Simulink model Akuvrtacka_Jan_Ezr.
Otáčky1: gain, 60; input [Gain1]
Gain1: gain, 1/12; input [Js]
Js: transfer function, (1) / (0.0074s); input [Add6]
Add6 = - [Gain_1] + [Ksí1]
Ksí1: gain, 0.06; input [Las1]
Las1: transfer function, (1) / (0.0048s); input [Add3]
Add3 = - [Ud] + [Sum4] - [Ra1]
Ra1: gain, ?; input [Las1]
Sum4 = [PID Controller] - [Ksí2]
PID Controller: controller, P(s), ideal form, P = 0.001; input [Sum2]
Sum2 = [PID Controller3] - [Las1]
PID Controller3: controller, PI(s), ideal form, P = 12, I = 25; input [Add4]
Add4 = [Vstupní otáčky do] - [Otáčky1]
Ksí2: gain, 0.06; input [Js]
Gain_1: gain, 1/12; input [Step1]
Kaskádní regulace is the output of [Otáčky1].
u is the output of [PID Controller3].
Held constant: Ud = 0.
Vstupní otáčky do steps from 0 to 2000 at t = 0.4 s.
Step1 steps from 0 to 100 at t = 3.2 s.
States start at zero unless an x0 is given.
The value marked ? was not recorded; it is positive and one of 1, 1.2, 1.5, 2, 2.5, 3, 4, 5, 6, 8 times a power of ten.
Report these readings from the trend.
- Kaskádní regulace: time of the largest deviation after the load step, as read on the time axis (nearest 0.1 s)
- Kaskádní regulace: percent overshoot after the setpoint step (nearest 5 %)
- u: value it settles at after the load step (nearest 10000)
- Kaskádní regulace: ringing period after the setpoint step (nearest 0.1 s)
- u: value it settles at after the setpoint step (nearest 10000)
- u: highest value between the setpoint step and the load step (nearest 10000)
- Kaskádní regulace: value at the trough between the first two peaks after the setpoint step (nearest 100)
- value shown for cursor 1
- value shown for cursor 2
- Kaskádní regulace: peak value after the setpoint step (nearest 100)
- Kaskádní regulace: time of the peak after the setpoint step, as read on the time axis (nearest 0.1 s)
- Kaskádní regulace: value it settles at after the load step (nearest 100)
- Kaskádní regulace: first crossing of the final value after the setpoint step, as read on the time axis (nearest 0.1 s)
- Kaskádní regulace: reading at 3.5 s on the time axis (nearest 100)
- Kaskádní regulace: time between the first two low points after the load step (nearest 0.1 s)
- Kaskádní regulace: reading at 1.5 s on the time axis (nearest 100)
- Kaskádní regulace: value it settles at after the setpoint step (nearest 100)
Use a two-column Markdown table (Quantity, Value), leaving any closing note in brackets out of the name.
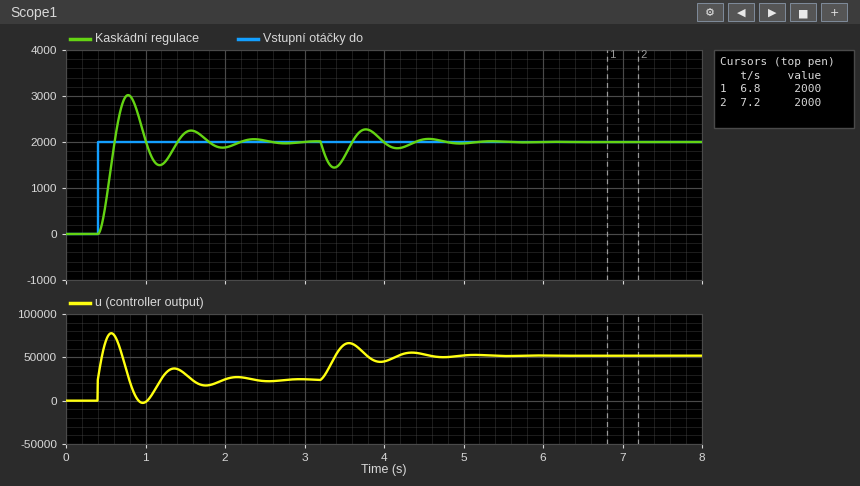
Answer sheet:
| Quantity | Value |
|---|---|
| Kaskádní regulace: time of the largest deviation after the load step, as read on the time axis | 3.4 s |
| Kaskádní regulace: percent overshoot after the setpoint step | 50 % |
| u: value it settles at after the load step | 50000 |
| Kaskádní regulace: ringing period after the setpoint step | 0.8 s |
| u: value it settles at after the setpoint step | 20000 |
| u: highest value between the setpoint step and the load step | 80000 |
| Kaskádní regulace: value at the trough between the first two peaks after the setpoint step | 1500 |
| value shown for cursor 1 | 2000 |
| value shown for cursor 2 | 2000 |
| Kaskádní regulace: peak value after the setpoint step | 3000 |
| Kaskádní regulace: time of the peak after the setpoint step, as read on the time axis | 0.8 s |
| Kaskádní regulace: value it settles at after the load step | 2000 |
| Kaskádní regulace: first crossing of the final value after the setpoint step, as read on the time axis | 0.6 s |
| Kaskádní regulace: reading at 3.5 s on the time axis | 1700 |
| Kaskádní regulace: time between the first two low points after the load step | 0.8 s |
| Kaskádní regulace: reading at 1.5 s on the time axis | 2200 |
| Kaskádní regulace: value it settles at after the setpoint step | 2000 |
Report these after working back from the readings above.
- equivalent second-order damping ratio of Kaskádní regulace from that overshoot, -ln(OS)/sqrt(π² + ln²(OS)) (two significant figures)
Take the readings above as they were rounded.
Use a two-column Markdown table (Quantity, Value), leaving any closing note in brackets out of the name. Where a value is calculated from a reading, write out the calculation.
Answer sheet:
| Quantity | Value |
|---|---|
| equivalent second-order damping ratio of Kaskádní regulace from that overshoot, -ln(OS)/sqrt(π² + ln²(OS)) | ln(0.5) = -0.693; 0.693 / sqrt(9.870 + 0.480) = 0.22 |
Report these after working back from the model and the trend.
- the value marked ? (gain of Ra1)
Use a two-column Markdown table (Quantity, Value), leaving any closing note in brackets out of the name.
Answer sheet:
| Quantity | Value |
|---|---|
| the value marked ? | 0.2 |
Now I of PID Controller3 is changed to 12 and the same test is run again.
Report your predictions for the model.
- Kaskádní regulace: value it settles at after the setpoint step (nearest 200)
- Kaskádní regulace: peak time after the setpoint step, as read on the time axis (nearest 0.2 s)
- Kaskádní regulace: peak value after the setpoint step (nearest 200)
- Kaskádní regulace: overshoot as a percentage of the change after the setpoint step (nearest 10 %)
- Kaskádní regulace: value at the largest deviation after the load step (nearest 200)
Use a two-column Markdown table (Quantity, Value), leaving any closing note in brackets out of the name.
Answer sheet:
| Quantity | Value |
|---|---|
| Kaskádní regulace: value it settles at after the setpoint step | 2000 |
| Kaskádní regulace: peak time after the setpoint step, as read on the time axis | 1.0 s |
| Kaskádní regulace: peak value after the setpoint step | 2600 |
| Kaskádní regulace: overshoot as a percentage of the change after the setpoint step | 30 % |
| Kaskádní regulace: value at the largest deviation after the load step | 1400 |
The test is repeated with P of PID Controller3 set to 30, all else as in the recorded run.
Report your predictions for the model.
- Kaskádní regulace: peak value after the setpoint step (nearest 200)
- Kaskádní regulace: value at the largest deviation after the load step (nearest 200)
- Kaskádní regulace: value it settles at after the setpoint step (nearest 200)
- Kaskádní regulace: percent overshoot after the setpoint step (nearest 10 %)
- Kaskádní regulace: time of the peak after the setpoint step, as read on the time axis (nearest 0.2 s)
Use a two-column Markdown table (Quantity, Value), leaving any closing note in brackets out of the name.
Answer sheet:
| Quantity | Value |
|---|---|
| Kaskádní regulace: peak value after the setpoint step | 3200 |
| Kaskádní regulace: value at the largest deviation after the load step | 1600 |
| Kaskádní regulace: value it settles at after the setpoint step | 2000 |
| Kaskádní regulace: percent overshoot after the setpoint step | 60 % |
| Kaskádní regulace: time of the peak after the setpoint step, as read on the time axis | 0.6 s |
